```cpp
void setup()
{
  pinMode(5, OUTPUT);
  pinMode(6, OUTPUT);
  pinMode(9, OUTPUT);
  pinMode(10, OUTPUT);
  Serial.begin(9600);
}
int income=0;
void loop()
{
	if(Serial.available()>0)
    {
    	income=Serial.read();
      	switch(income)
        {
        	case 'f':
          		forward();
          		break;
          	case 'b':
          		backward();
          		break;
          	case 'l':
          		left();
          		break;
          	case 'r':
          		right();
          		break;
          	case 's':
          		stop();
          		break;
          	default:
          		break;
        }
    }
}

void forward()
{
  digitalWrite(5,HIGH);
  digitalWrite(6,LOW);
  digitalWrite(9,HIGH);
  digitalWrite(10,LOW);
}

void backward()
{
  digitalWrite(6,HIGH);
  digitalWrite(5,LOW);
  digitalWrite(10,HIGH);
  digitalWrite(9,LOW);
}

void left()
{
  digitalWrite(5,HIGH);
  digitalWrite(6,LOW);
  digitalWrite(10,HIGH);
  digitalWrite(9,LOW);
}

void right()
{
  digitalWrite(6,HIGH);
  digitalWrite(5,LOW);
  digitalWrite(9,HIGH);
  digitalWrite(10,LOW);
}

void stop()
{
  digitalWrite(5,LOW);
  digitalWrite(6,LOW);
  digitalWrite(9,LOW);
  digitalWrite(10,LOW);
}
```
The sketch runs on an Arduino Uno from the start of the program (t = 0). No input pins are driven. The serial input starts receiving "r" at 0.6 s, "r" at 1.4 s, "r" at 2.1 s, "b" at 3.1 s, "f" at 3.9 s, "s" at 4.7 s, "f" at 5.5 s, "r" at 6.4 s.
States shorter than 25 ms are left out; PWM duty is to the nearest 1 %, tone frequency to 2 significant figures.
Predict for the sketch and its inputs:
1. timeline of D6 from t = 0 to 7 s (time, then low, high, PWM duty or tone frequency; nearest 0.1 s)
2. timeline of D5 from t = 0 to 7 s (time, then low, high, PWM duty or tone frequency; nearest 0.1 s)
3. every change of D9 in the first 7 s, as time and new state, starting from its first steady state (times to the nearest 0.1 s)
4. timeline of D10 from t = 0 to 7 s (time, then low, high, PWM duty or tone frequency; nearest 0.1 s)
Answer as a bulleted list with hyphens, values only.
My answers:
- 0 s low; 0.6 s high; 3.9 s low; 6.4 s high
- 0 s low; 3.9 s high; 4.7 s low; 5.5 s high; 6.4 s low
- 0 s low; 0.6 s high; 3.1 s low; 3.9 s high; 4.7 s low; 5.5 s high
- 0 s low; 3.1 s high; 3.9 s low
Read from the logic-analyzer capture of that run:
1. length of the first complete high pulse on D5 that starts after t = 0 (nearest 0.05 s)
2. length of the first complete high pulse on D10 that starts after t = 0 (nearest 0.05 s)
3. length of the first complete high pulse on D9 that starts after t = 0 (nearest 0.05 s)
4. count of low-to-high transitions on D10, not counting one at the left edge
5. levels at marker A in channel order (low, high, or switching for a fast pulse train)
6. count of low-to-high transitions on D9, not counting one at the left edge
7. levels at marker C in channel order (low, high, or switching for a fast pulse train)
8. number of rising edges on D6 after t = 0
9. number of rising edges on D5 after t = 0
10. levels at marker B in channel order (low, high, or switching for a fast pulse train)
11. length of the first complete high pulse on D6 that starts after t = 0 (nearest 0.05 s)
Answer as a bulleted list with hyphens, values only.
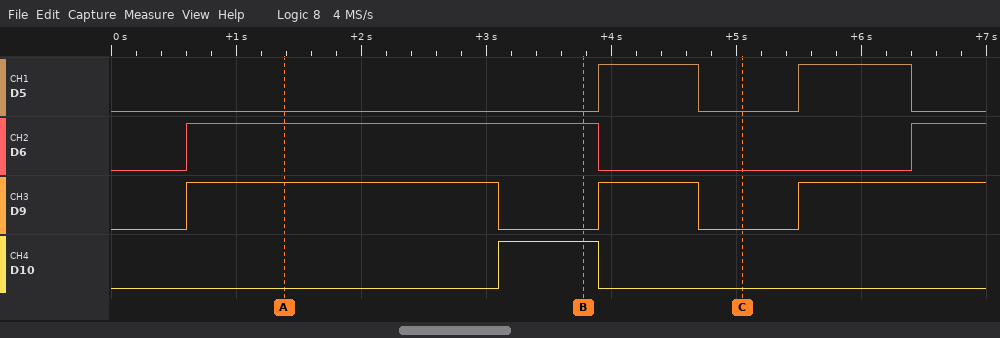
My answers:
- 0.80 s
- 0.80 s
- 2.50 s
- 1
- D5 low, D6 high, D9 high, D10 low
- 3
- D5 low, D6 low, D9 low, D10 low
- 2
- 2
- D5 low, D6 high, D9 low, D10 high
- 3.30 s
